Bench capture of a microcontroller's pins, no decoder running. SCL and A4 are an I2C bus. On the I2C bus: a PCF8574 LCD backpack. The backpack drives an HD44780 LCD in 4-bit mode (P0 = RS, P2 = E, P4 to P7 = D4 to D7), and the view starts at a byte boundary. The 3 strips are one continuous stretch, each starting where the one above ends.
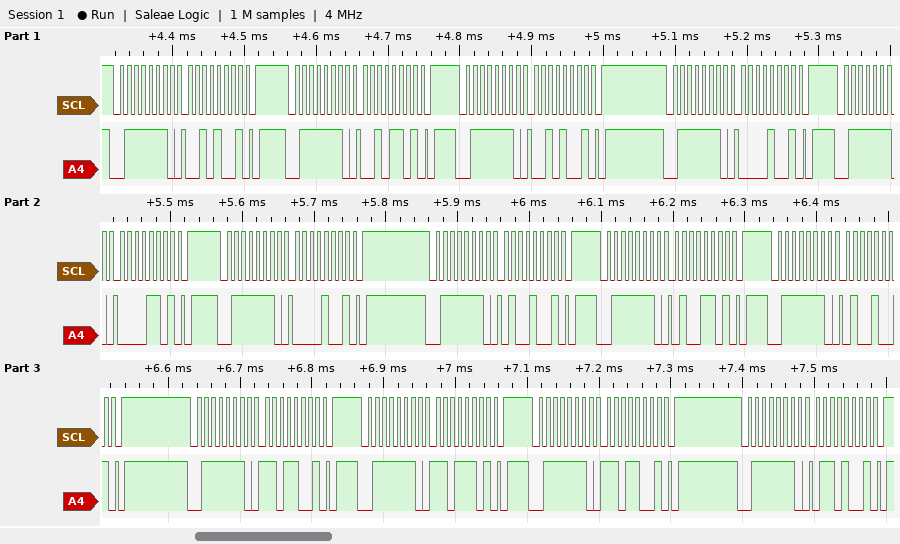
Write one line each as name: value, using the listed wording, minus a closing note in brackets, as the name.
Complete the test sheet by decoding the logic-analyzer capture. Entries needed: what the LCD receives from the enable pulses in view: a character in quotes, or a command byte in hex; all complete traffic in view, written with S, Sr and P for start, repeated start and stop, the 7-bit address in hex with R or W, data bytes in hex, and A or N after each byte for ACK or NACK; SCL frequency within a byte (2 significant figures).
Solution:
what the LCD receives from the enable pulses in view: a character in quotes, or a command byte in hex: ' ' 'M'
all complete traffic in view, written with S, Sr and P for start, repeated start and stop, the 7-bit address in hex with R or W, data bytes in hex, and A or N after each byte for ACK or NACK: S 3FW A 29 A P S 3FW A 2D A P S 3FW A 29 A P S 3FW A 09 A P S 3FW A 0D A P S 3FW A 09 A P S 3FW A 49 A P S 3FW A 4D A P S 3FW A 49 A P S 3FW A D9 A P S 3FW A DD A P S 3FW A D9 A P S 3FW A 69 A P
SCL frequency within a byte: 100 kHz
